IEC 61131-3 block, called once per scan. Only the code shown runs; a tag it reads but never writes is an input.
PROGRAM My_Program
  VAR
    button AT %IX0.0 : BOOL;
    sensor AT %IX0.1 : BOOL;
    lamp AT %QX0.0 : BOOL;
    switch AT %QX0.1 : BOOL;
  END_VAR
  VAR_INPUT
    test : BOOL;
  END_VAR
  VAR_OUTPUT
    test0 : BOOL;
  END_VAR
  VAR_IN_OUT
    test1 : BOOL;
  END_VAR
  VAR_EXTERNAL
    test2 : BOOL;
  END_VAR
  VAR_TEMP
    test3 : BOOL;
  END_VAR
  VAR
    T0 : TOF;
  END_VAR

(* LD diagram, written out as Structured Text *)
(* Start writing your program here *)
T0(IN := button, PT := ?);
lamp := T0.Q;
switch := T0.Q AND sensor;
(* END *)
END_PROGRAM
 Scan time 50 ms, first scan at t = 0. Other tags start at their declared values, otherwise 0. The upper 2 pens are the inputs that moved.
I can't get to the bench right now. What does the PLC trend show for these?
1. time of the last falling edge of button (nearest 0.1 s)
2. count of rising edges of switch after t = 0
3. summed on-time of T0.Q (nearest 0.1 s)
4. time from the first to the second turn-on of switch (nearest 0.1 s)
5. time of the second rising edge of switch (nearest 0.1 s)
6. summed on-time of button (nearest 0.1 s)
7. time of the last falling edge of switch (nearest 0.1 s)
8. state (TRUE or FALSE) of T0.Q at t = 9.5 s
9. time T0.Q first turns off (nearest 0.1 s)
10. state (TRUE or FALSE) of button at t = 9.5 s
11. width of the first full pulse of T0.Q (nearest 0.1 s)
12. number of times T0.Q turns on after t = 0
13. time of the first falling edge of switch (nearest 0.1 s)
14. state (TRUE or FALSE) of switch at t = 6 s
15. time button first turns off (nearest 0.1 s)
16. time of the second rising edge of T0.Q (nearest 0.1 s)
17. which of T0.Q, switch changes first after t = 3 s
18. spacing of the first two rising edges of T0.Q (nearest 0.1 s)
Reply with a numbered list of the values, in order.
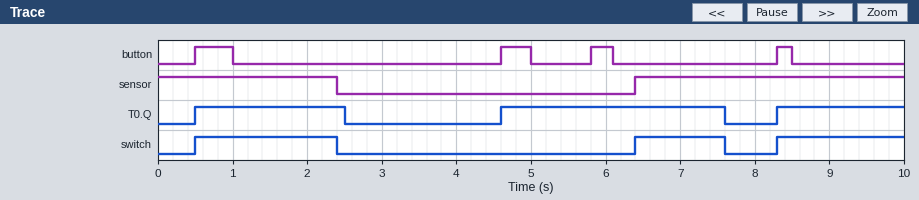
1. 8.5 s
2. 3
3. 6.7 s
4. 5.9 s
5. 6.4 s
6. 1.4 s
7. 7.6 s
8. TRUE
9. 2.5 s
10. FALSE
11. 2.0 s
12. 3
13. 2.4 s
14. FALSE
15. 1.0 s
16. 4.6 s
17. T0.Q
18. 4.1 s
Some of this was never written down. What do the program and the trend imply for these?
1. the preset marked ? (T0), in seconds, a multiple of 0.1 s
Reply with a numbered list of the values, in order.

1. 1.5 s
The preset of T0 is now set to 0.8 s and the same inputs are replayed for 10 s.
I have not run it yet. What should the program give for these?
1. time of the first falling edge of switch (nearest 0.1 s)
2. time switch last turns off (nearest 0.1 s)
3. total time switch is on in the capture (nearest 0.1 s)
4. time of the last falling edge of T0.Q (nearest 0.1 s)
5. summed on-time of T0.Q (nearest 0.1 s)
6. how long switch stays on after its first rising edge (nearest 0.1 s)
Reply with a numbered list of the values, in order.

1. 1.8 s
2. 9.3 s
3. 2.8 s
4. 9.3 s
5. 4.6 s
6. 1.3 s
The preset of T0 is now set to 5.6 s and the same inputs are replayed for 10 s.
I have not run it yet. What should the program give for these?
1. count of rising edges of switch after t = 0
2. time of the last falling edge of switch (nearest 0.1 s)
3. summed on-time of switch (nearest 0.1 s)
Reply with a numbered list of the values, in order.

1. 2
2. 2.4 s
3. 5.5 s
